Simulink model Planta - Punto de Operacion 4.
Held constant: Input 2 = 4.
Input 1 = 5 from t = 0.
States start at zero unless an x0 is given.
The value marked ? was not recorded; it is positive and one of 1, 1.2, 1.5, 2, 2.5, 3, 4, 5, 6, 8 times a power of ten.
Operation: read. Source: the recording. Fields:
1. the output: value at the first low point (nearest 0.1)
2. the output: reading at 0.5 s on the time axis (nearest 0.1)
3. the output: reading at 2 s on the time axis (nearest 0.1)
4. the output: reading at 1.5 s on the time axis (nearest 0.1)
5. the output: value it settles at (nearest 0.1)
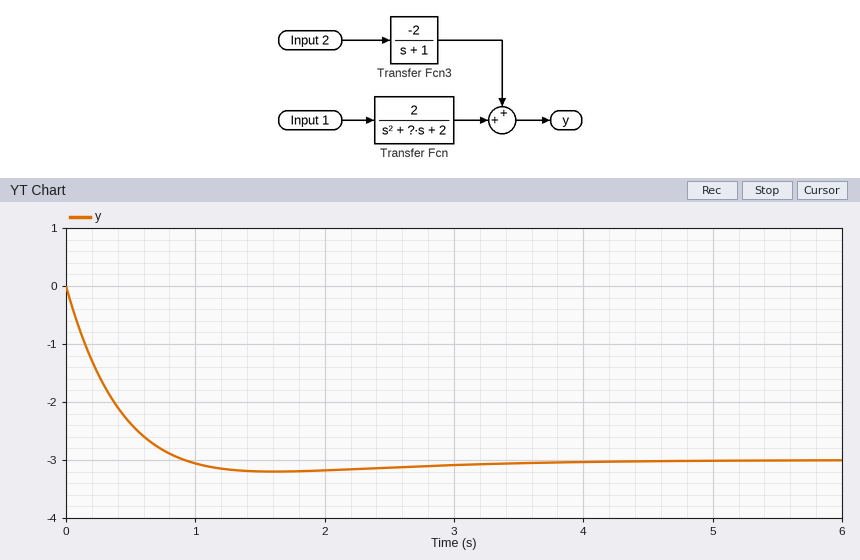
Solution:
-3.2
-2.4
-3.2
-3.2
-3.0
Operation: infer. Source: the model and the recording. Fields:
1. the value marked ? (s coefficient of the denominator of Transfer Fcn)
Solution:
3
